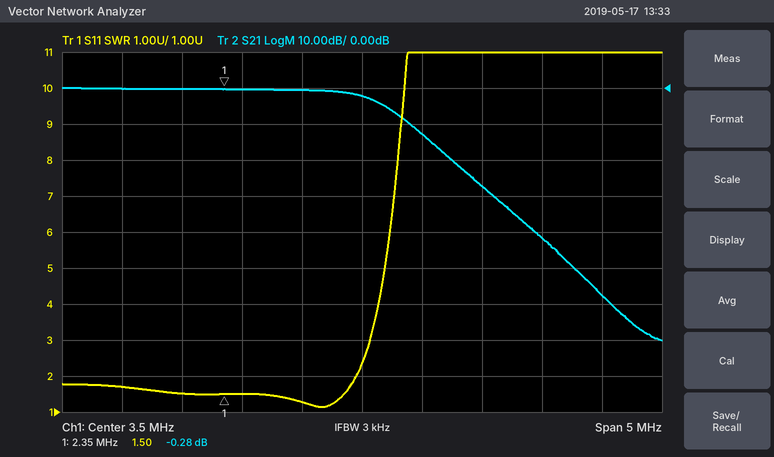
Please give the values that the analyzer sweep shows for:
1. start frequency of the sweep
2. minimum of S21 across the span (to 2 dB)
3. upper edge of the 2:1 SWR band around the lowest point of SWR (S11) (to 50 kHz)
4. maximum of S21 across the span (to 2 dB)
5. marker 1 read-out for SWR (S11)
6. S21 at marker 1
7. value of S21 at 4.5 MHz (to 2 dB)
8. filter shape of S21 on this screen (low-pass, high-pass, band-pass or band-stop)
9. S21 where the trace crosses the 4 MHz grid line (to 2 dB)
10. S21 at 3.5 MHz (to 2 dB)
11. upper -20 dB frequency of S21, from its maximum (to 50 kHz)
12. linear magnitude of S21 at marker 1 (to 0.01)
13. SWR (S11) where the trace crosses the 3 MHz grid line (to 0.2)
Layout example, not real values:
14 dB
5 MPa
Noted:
1 MHz
-70 dB
3.45 MHz
0 dB
1.50
-0.28 dB
-28 dB
low-pass
-12 dB
-2 dB
4.25 MHz
0.97
1.2
